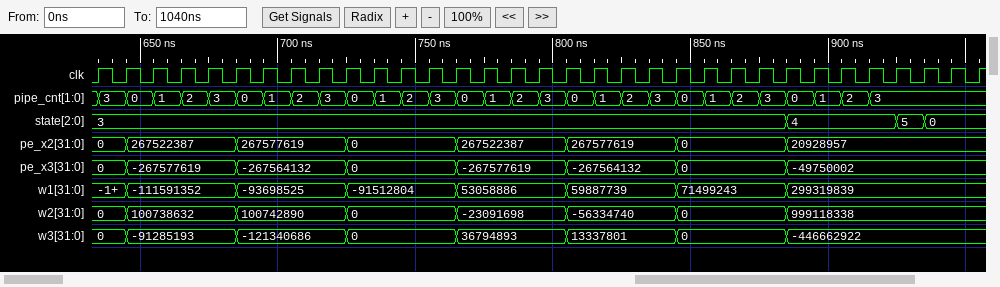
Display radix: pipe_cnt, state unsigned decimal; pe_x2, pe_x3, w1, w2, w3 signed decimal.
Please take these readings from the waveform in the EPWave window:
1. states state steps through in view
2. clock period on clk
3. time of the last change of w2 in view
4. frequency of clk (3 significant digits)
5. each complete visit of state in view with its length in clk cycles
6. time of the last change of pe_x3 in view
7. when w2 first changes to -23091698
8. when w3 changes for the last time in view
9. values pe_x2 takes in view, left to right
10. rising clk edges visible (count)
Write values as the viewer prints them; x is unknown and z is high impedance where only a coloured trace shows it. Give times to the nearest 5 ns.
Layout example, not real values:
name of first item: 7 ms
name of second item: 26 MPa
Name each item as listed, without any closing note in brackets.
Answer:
states state steps through in view: 3, 4, 5, 0
clock period on clk: 10 ns
time of the last change of w2 in view: 885 ns
frequency of clk: 100 MHz
each complete visit of state in view with its length in clk cycles: 4: 4, 5: 1
time of the last change of pe_x3 in view: 885 ns
when w2 first changes to -23091698: 765 ns
when w3 changes for the last time in view: 885 ns
values pe_x2 takes in view, left to right: 0, 267522387, 267577619, 0, 267522387, 267577619, 0, 20928957
rising clk edges visible: 33
